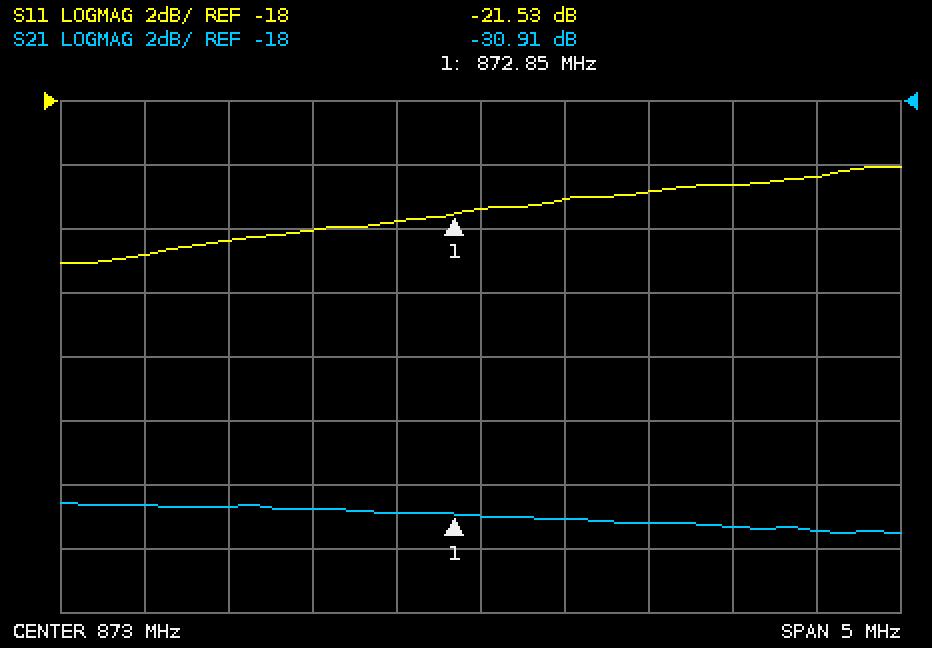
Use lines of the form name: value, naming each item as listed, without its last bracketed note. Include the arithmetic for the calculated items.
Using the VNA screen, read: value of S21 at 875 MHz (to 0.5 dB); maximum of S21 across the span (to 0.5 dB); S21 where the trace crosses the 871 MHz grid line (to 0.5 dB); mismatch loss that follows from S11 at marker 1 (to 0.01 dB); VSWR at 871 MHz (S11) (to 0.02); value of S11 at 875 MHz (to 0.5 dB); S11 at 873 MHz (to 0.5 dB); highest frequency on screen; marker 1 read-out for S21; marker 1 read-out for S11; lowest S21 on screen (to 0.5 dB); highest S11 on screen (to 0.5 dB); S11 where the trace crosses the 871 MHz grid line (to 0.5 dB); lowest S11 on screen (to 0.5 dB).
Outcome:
value of S21 at 875 MHz: -31.5 dB
maximum of S21 across the span: -30.5 dB
S21 where the trace crosses the 871 MHz grid line: -30.5 dB
mismatch loss that follows from S11 at marker 1: −10 log10(1 − 10^(-21.53/10)) ≈ 0.03 dB
VSWR at 871 MHz (S11): |Γ| = 10^(-23/20) = 0.0708; VSWR = (1 + 0.0708)/(1 − 0.0708) ≈ 1.15, so 1.16 to the nearest 0.02
value of S11 at 875 MHz: -20.5 dB
S11 at 873 MHz: -21.5 dB
highest frequency on screen: 875.5 MHz
marker 1 read-out for S21: -30.91 dB
marker 1 read-out for S11: -21.53 dB
lowest S21 on screen: -31.5 dB
highest S11 on screen: -20.0 dB
S11 where the trace crosses the 871 MHz grid line: -23.0 dB
lowest S11 on screen: -23.0 dB
